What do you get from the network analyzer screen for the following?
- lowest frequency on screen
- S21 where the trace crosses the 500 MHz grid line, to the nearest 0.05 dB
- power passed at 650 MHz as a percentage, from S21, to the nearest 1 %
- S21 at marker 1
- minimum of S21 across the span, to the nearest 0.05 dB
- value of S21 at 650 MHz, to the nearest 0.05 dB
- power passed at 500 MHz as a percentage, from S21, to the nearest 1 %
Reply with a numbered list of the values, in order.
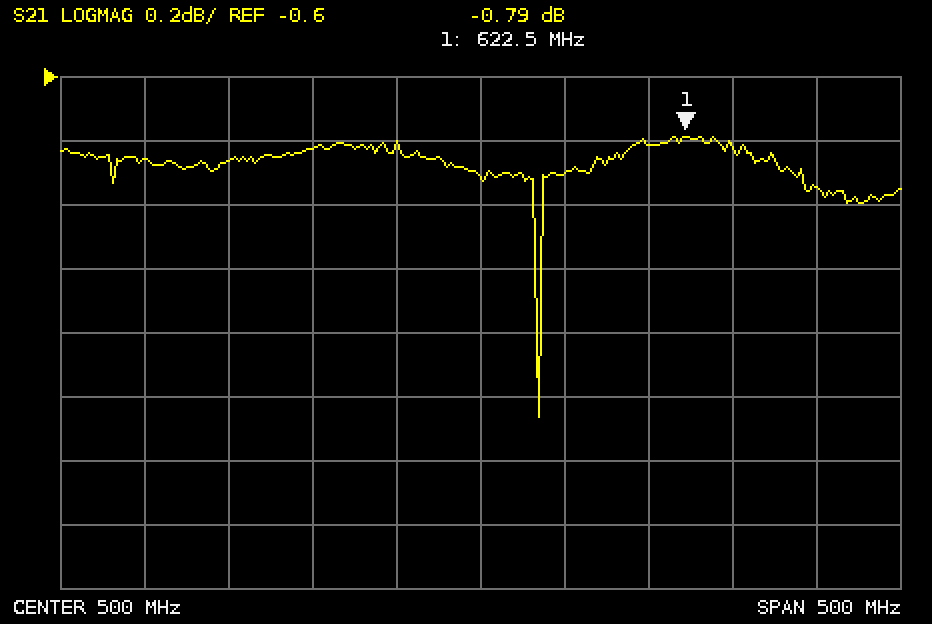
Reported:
1. 250 MHz
2. -0.90 dB
3. 83 %
4. -0.79 dB
5. -1.65 dB
6. -0.80 dB
7. 81 %
